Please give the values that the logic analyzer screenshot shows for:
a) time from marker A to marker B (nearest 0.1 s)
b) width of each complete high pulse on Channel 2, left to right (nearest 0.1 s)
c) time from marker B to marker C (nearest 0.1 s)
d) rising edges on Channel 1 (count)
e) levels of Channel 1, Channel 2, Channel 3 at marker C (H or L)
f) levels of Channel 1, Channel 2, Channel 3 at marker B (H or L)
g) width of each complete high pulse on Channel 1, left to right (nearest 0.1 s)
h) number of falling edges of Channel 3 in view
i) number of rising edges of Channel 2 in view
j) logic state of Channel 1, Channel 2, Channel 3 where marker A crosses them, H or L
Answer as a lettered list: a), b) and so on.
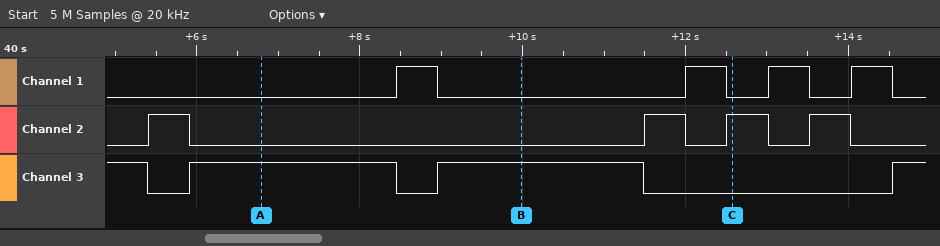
a) 3.2 s
b) 0.5 s, 0.5 s, 0.5 s, 0.5 s
c) 2.6 s
d) 4
e) Channel 1=L, Channel 2=H, Channel 3=L
f) Channel 1=L, Channel 2=L, Channel 3=H
g) 0.5 s, 0.5 s, 0.5 s, 0.5 s
h) 3
i) 4
j) Channel 1=L, Channel 2=L, Channel 3=H
